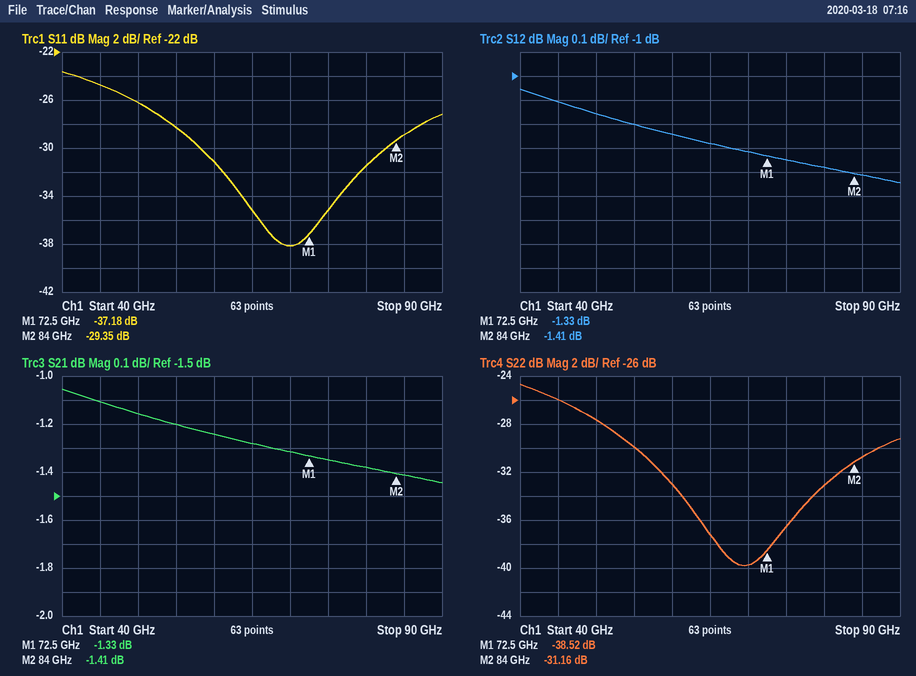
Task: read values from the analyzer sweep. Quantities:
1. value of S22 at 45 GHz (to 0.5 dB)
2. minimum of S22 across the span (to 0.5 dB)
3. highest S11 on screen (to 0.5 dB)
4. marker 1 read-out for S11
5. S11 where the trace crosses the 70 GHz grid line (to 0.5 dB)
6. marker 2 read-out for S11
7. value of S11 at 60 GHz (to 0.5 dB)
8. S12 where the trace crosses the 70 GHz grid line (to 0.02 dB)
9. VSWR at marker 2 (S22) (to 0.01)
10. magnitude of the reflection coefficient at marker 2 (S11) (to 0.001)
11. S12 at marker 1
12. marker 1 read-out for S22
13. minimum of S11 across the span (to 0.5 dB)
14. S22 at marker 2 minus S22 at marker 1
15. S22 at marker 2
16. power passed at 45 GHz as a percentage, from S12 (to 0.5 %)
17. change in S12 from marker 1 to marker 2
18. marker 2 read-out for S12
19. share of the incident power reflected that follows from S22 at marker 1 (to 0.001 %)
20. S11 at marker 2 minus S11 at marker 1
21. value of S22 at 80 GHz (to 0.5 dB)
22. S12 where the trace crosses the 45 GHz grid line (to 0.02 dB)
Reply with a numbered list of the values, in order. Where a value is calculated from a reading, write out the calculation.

1. -26.0 dB
2. -40.0 dB
3. -23.5 dB
4. -37.18 dB
5. -38.0 dB
6. -29.35 dB
7. -31.0 dB
8. -1.32 dB
9. (1 + 0.0277)/(1 − 0.0277) ≈ 1.06
10. 10^(-29.35/20) ≈ 0.034
11. -1.33 dB
12. -38.52 dB
13. -38.0 dB
14. -31.16 − (-38.52) = 7.36 dB
15. -31.16 dB
16. 10^(-1.1/10) ≈ 77.6 %, so 77.5 % to the nearest 0.5 %
17. -1.41 − (-1.33) = -0.08 dB
18. -1.41 dB
19. 10^(-38.52/10) ≈ 0.014 %
20. -29.35 − (-37.18) = 7.83 dB
21. -33.0 dB
22. -1.10 dB
